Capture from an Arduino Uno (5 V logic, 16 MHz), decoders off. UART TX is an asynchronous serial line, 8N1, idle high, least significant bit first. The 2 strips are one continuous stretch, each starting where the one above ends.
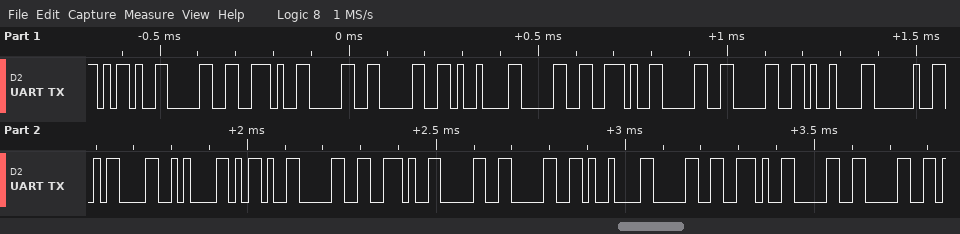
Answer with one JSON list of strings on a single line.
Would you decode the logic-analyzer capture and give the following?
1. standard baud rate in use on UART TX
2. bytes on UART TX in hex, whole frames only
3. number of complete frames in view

["57600 baud", "2D 30 2E 30 30 09 30 2E 30 30 09 20 0D 0A 2D 30 2E 30 30 09 30 2E 30 30", "24"]
